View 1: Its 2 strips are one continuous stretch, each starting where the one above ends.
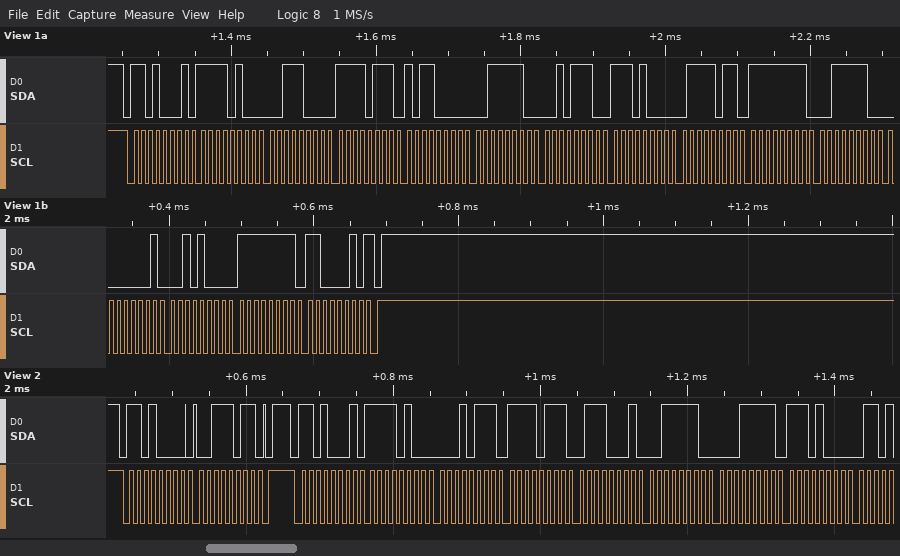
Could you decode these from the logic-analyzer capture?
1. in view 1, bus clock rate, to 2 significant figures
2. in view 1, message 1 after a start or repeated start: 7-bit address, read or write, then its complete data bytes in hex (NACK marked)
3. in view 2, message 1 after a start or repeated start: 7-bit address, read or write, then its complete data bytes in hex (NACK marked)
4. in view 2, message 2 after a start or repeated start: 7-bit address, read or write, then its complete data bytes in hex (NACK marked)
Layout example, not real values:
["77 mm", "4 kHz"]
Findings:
["100 kHz", "0x68 read: F4 38 F7 B0 3E 2E E8 7B FF 3E 01 28 FF C2 NACK", "0x68 write: 3B", "0x68 read: F4 17 F7 71 3E 1F E8"]
